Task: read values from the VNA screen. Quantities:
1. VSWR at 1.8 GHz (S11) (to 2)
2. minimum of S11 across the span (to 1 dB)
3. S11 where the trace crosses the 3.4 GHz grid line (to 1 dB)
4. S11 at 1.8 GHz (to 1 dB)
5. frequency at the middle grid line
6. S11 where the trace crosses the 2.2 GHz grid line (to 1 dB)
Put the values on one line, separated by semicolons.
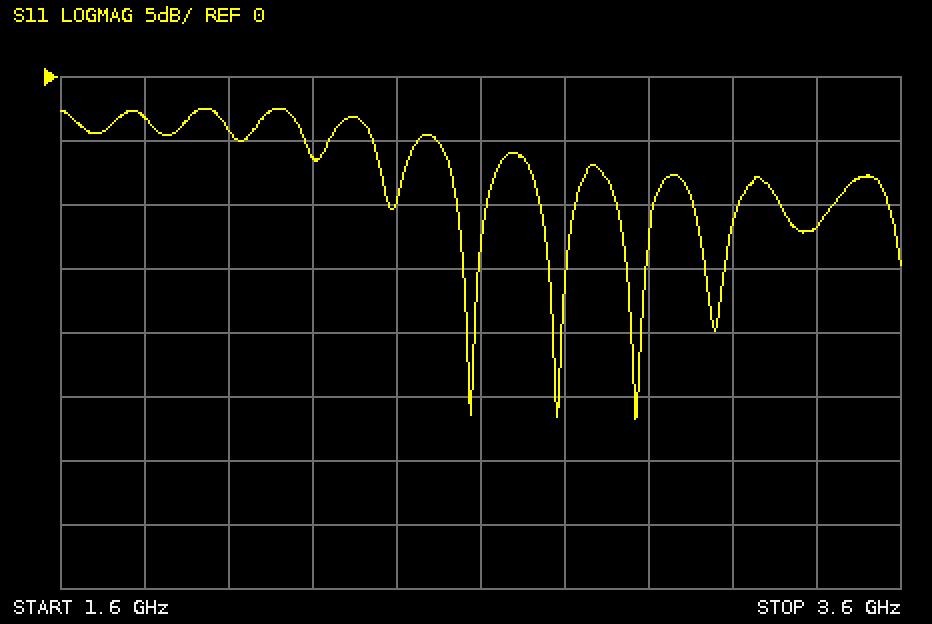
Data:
6; -27 dB; -12 dB; -3 dB; 2.6 GHz; -6 dB
